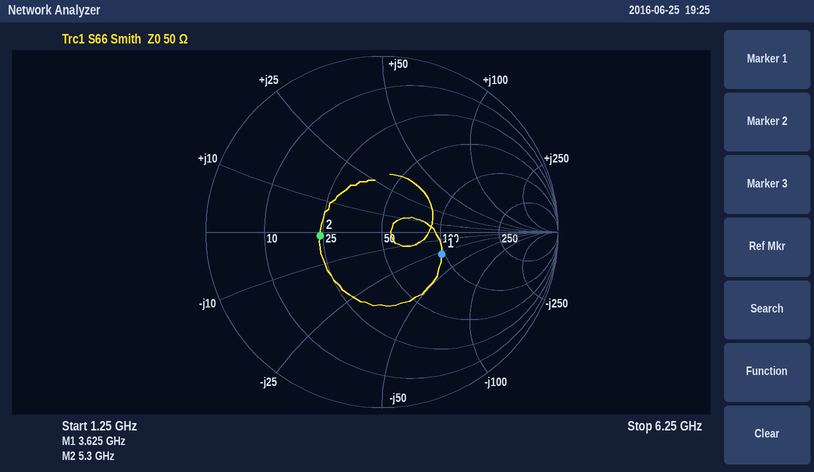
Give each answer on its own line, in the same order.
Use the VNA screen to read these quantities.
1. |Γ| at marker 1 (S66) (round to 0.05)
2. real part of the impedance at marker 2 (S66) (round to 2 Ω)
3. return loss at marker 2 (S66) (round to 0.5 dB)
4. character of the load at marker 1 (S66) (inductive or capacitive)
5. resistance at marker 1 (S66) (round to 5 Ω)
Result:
0.35
24 Ω
9.0 dB
capacitive
95 Ω
